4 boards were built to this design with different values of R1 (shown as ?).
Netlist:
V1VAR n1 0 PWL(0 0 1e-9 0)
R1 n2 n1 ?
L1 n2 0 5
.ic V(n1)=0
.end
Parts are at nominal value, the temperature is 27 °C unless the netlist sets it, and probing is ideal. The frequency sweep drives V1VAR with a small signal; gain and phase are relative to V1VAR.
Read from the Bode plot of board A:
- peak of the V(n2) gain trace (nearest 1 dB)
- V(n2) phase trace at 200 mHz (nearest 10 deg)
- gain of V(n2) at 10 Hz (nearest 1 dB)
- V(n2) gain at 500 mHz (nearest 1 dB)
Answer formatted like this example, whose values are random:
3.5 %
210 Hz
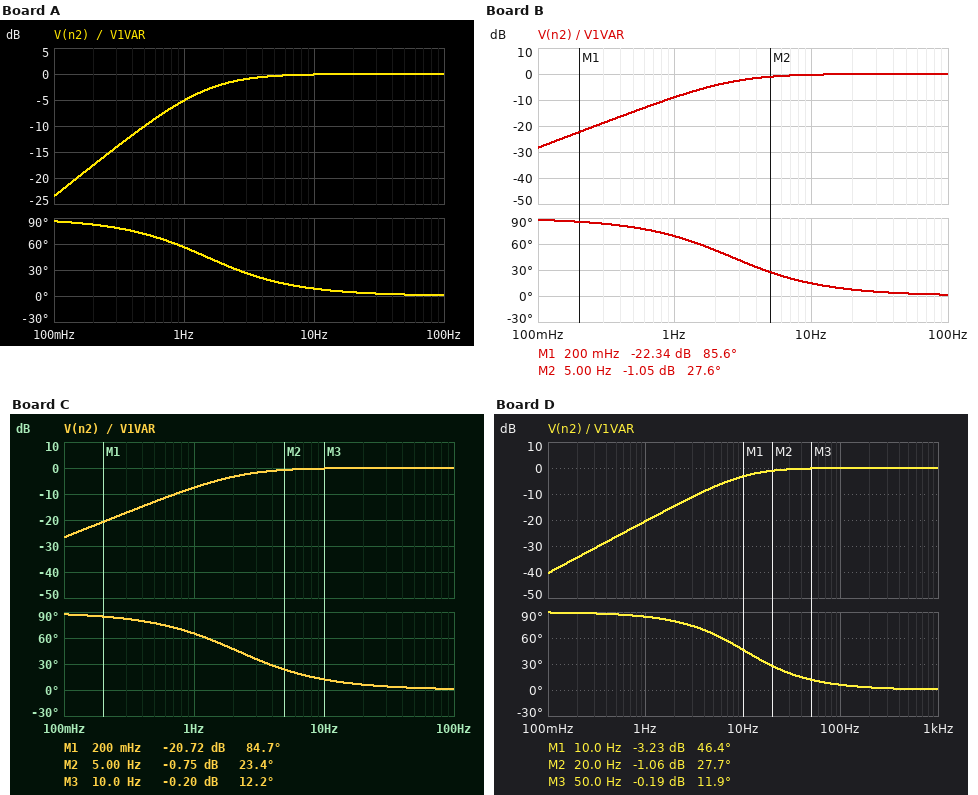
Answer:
0 dB
80 deg
0 dB
-10 dB
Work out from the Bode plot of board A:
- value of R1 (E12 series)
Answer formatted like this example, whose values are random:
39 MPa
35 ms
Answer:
47 Ω
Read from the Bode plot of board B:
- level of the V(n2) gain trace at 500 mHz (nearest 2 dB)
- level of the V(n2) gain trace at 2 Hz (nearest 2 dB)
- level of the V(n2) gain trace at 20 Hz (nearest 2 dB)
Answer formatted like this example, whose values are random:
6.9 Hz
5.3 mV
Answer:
-14 dB
-4 dB
0 dB
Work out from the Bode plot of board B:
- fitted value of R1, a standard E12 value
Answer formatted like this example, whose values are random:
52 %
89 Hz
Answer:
82 Ω
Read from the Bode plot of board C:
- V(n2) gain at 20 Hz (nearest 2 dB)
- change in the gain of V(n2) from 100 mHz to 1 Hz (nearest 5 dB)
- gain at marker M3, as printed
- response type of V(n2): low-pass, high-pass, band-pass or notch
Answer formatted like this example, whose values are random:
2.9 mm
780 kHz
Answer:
0 dB
20 dB
-0.20 dB
high-pass
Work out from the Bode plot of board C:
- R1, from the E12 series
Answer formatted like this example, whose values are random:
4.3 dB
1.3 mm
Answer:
68 Ω
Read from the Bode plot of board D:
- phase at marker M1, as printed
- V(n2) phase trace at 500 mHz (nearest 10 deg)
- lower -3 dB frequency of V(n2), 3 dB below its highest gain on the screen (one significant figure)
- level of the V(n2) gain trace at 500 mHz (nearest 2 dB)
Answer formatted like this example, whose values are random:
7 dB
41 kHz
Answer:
46.4 deg
90 deg
10 Hz
-26 dB
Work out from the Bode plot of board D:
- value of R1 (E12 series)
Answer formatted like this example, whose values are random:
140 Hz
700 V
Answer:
330 Ω
